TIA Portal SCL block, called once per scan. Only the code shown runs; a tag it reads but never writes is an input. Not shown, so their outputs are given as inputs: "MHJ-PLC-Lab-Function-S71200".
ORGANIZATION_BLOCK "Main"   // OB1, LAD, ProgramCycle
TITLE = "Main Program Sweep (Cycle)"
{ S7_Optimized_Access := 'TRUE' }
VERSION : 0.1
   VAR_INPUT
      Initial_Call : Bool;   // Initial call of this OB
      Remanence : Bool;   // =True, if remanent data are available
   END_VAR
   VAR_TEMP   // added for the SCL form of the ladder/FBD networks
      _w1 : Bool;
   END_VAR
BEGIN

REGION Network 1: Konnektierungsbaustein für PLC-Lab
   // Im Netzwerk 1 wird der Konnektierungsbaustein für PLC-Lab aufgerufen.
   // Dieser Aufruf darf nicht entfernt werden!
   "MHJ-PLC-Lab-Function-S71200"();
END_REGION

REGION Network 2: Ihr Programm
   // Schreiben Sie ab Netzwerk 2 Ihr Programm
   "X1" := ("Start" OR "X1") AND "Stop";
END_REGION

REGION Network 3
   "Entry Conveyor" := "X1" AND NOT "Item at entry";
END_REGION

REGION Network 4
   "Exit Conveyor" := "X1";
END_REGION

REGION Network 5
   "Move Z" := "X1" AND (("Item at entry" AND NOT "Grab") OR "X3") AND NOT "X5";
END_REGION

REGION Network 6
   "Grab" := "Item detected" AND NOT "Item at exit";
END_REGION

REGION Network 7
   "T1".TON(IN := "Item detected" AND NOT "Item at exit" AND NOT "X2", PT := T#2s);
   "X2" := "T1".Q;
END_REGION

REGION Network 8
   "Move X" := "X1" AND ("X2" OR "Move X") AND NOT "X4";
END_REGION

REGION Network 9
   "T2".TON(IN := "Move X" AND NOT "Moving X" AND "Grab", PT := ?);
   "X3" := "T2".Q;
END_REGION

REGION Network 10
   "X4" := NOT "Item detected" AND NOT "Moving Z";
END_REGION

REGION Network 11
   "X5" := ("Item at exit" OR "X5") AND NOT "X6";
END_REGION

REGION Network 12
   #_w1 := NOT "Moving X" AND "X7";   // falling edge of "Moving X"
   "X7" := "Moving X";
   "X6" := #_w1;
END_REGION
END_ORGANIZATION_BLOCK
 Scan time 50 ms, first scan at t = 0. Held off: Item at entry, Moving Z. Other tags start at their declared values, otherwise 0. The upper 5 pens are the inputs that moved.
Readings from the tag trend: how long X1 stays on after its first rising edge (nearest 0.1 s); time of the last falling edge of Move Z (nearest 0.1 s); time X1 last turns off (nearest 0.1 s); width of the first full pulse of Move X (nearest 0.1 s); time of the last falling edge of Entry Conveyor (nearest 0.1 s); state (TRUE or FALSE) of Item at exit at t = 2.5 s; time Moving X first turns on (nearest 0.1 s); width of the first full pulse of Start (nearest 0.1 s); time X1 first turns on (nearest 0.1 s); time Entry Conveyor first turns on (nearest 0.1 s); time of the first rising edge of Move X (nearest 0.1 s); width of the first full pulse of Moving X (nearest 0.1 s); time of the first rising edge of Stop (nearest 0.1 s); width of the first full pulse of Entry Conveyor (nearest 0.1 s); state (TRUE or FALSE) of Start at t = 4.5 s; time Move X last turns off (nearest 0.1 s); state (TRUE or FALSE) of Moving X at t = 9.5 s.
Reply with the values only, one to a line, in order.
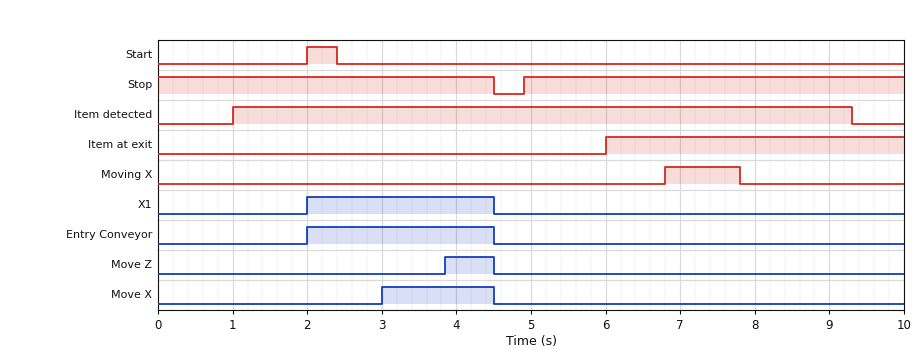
2.5 s
4.5 s
4.5 s
1.5 s
4.5 s
FALSE
6.8 s
0.4 s
2.0 s
2.0 s
3.0 s
1.0 s
4.9 s
2.5 s
FALSE
4.5 s
FALSE
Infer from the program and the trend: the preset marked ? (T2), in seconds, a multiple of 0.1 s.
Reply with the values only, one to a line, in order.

0.8 s
